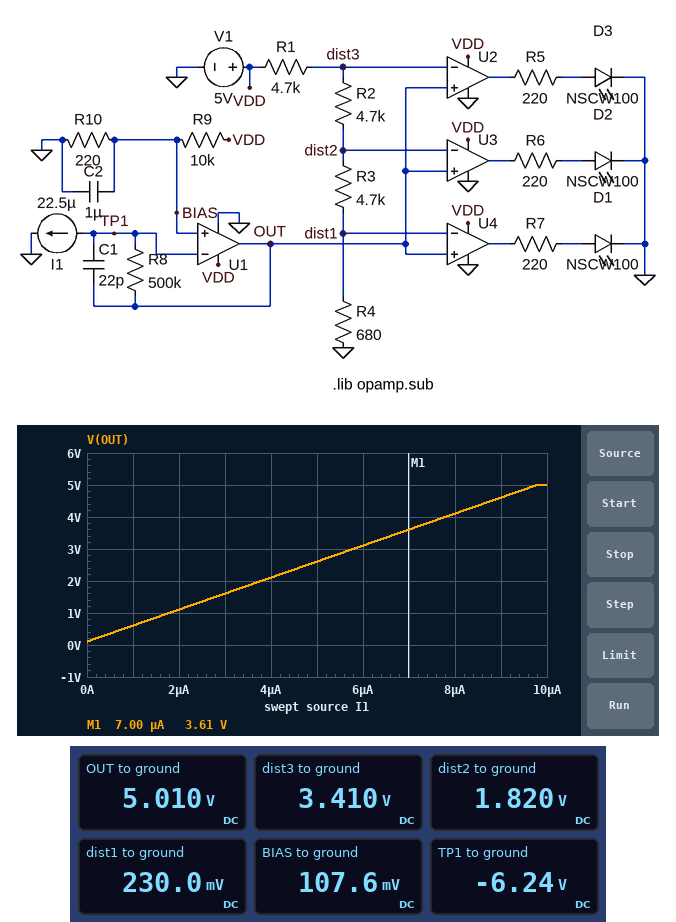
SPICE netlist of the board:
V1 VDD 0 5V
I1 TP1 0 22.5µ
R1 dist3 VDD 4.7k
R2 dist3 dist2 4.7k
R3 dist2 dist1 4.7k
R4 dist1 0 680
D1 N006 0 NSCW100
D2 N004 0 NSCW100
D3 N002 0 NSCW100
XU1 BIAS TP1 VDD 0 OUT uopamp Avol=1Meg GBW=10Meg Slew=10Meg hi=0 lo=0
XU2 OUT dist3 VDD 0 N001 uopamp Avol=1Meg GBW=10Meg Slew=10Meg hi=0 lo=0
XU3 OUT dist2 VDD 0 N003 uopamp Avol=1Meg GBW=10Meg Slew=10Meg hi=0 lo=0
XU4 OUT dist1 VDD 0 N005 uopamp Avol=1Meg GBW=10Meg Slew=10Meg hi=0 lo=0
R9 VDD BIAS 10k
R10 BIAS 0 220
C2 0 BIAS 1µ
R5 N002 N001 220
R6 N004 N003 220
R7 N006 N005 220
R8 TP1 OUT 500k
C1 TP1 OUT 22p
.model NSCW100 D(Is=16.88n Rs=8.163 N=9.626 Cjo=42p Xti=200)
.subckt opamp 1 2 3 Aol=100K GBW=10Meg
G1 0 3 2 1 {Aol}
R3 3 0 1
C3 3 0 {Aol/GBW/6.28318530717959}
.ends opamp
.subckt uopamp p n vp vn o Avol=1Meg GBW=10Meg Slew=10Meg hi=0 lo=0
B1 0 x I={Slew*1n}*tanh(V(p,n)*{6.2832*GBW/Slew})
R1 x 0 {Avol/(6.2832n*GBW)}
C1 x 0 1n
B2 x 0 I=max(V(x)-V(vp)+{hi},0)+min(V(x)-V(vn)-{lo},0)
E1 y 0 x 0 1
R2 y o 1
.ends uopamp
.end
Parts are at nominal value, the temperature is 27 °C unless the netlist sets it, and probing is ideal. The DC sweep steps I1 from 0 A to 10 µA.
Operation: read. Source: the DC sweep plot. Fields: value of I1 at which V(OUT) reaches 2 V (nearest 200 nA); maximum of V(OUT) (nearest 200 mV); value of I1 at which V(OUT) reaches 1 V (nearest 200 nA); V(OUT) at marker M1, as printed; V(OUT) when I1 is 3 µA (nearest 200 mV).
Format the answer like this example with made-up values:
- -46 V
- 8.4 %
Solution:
- 3.8 µA
- 5.0 V
- 1.8 µA
- 3.61 V
- 1.6 V
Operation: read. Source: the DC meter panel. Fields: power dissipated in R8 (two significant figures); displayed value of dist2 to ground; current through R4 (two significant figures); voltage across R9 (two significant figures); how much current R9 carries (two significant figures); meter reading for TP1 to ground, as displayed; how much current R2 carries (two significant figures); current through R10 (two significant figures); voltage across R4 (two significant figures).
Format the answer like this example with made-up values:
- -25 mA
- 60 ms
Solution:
- 250 µW
- 1.820 V
- 340 µA
- 4.9 V
- 490 µA
- -6.24 V
- 340 µA
- 490 µA
- 230 mV
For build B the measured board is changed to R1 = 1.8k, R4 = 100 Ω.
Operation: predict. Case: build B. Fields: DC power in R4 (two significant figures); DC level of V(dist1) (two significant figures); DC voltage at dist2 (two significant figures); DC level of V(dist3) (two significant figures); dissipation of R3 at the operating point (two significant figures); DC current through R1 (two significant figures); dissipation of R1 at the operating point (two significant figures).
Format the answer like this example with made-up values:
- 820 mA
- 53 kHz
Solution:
- 20 µW
- 44 mV
- 2.1 V
- 4.2 V
- 920 µW
- 440 µA
- 350 µW
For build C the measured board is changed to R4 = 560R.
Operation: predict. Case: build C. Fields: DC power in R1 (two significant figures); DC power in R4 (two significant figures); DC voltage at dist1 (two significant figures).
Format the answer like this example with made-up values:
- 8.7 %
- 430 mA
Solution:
- 550 µW
- 65 µW
- 190 mV
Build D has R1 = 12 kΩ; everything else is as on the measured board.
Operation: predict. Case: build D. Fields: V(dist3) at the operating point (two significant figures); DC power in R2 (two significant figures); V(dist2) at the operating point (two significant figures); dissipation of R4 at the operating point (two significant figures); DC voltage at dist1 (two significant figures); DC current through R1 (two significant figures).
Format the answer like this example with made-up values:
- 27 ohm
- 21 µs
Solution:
- 2.3 V
- 240 µW
- 1.2 V
- 35 µW
- 150 mV
- 230 µA
